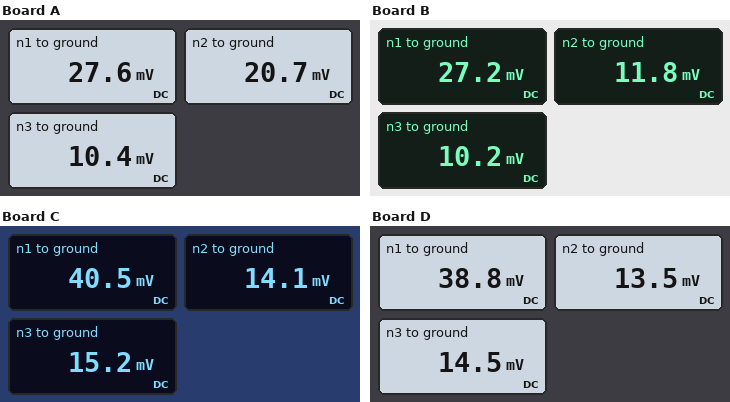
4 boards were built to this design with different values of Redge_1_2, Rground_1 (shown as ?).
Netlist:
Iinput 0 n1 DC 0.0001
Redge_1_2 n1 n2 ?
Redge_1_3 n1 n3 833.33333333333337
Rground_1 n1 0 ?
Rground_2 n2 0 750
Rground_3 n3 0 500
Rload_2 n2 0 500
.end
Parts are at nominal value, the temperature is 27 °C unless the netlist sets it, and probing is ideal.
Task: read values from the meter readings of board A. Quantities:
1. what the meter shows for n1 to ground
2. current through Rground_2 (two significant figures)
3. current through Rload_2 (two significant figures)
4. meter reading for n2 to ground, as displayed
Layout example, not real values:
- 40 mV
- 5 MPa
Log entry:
- 27.6 mV
- 28 µA
- 41 µA
- 20.7 mV
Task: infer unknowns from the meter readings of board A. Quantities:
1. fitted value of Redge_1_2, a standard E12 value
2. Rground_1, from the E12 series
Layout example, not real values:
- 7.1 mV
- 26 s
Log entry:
- 100 Ω
- 2.7 kΩ
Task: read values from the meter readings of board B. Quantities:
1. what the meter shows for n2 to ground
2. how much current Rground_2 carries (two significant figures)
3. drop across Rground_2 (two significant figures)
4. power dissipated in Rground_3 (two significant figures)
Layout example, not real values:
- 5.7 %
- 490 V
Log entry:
- 11.8 mV
- 16 µA
- 12 mV
- 210 nW
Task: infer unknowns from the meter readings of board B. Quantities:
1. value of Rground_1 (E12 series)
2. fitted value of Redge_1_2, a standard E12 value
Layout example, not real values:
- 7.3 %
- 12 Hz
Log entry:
- 680 Ω
- 390 Ω
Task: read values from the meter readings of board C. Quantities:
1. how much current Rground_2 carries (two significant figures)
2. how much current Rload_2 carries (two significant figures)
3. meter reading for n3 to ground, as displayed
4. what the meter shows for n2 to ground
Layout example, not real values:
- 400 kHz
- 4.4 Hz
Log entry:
- 19 µA
- 28 µA
- 15.2 mV
- 14.1 mV
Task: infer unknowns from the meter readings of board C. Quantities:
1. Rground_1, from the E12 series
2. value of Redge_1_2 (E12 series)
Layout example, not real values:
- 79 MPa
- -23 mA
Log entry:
- 1.8 kΩ
- 560 Ω
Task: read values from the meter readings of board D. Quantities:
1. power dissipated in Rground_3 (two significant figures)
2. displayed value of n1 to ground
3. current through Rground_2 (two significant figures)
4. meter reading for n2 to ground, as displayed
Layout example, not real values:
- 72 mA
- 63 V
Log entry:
- 420 nW
- 38.8 mV
- 18 µA
- 13.5 mV
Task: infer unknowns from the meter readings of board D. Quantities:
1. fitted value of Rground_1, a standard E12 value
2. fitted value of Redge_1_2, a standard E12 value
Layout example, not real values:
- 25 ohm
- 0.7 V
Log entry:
- 1.5 kΩ
- 560 Ω
